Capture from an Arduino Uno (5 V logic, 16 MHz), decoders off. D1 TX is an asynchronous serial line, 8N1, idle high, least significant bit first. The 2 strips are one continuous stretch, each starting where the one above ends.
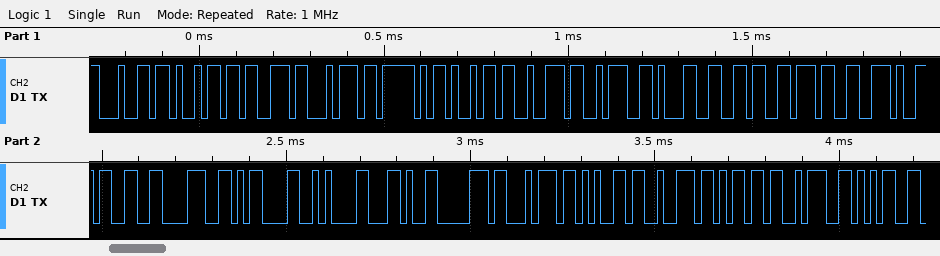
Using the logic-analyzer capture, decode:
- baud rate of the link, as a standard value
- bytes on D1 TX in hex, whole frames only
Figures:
57600 baud
0x64 0x69 0x73 0x74 0x5F 0x69 0x72 0x3A 0x31 0x36 0x37 0x2E 0x33 0x38 0x0D 0x0A 0x2C 0x70 0x74 0x65 0x72 0x6D 0x3A 0x35
